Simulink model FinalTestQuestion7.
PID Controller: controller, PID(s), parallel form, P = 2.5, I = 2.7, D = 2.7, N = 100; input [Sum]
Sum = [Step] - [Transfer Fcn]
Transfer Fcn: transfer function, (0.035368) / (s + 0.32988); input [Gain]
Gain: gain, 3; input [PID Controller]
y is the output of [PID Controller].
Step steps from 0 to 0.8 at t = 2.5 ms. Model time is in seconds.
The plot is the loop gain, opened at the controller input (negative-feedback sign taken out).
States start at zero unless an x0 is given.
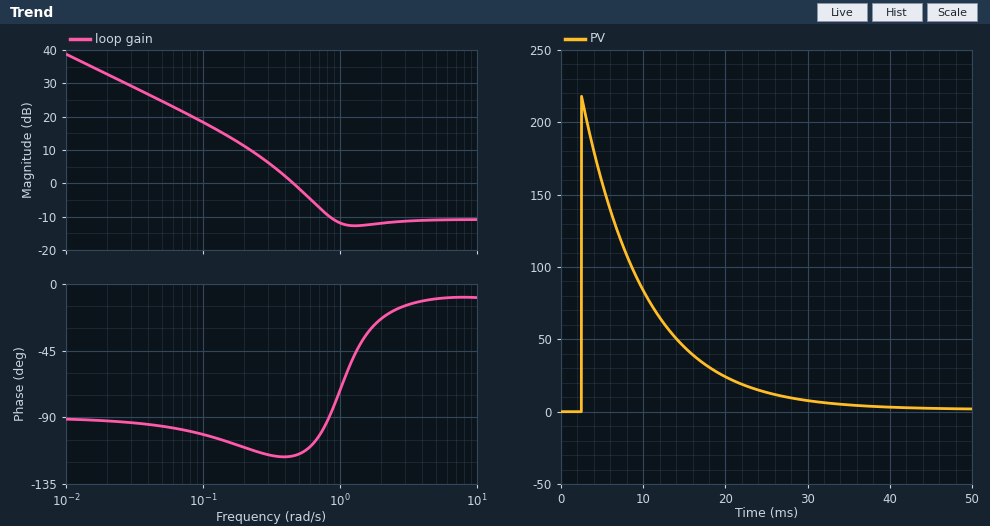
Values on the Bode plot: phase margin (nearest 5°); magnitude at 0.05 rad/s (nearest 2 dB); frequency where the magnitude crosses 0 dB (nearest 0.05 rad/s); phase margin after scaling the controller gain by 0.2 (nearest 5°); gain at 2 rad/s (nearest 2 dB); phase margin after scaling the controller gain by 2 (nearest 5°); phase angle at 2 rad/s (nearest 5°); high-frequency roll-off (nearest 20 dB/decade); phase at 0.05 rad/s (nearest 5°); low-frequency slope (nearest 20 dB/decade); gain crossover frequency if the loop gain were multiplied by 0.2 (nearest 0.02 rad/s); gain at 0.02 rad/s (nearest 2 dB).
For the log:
65°
24 dB
0.45 rad/s
75°
-12 dB
75°
-25°
0 dB/decade
-95°
-20 dB/decade
0.16 rad/s
32 dB
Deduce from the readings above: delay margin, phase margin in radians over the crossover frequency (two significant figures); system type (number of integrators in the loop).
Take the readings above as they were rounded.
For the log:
2.5 s
1
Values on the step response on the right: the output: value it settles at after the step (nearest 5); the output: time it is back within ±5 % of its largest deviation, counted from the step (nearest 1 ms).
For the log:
0
23 ms
